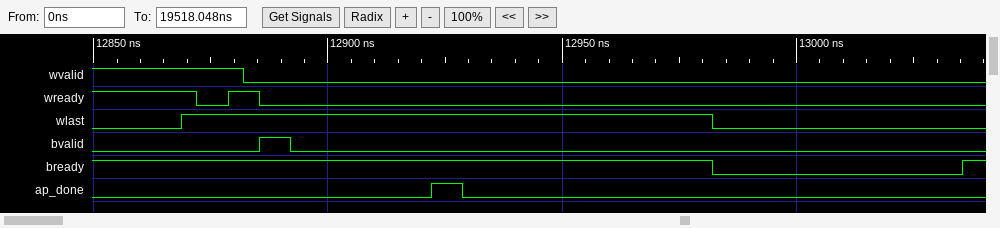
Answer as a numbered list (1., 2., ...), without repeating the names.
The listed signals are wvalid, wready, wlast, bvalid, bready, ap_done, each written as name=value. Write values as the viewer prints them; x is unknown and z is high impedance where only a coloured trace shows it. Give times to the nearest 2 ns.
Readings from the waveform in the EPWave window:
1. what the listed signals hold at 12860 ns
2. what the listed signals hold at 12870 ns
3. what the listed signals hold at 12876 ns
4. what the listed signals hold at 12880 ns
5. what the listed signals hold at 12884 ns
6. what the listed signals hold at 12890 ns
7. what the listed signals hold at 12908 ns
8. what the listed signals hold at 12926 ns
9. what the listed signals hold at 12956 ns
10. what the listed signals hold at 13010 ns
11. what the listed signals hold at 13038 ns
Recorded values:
1. wvalid=1, wready=1, wlast=0, bvalid=0, bready=1, ap_done=0
2. wvalid=1, wready=1, wlast=1, bvalid=0, bready=1, ap_done=0
3. wvalid=1, wready=0, wlast=1, bvalid=0, bready=1, ap_done=0
4. wvalid=1, wready=1, wlast=1, bvalid=0, bready=1, ap_done=0
5. wvalid=0, wready=1, wlast=1, bvalid=0, bready=1, ap_done=0
6. wvalid=0, wready=0, wlast=1, bvalid=1, bready=1, ap_done=0
7. wvalid=0, wready=0, wlast=1, bvalid=0, bready=1, ap_done=0
8. wvalid=0, wready=0, wlast=1, bvalid=0, bready=1, ap_done=1
9. wvalid=0, wready=0, wlast=1, bvalid=0, bready=1, ap_done=0
10. wvalid=0, wready=0, wlast=0, bvalid=0, bready=0, ap_done=0
11. wvalid=0, wready=0, wlast=0, bvalid=0, bready=1, ap_done=0
